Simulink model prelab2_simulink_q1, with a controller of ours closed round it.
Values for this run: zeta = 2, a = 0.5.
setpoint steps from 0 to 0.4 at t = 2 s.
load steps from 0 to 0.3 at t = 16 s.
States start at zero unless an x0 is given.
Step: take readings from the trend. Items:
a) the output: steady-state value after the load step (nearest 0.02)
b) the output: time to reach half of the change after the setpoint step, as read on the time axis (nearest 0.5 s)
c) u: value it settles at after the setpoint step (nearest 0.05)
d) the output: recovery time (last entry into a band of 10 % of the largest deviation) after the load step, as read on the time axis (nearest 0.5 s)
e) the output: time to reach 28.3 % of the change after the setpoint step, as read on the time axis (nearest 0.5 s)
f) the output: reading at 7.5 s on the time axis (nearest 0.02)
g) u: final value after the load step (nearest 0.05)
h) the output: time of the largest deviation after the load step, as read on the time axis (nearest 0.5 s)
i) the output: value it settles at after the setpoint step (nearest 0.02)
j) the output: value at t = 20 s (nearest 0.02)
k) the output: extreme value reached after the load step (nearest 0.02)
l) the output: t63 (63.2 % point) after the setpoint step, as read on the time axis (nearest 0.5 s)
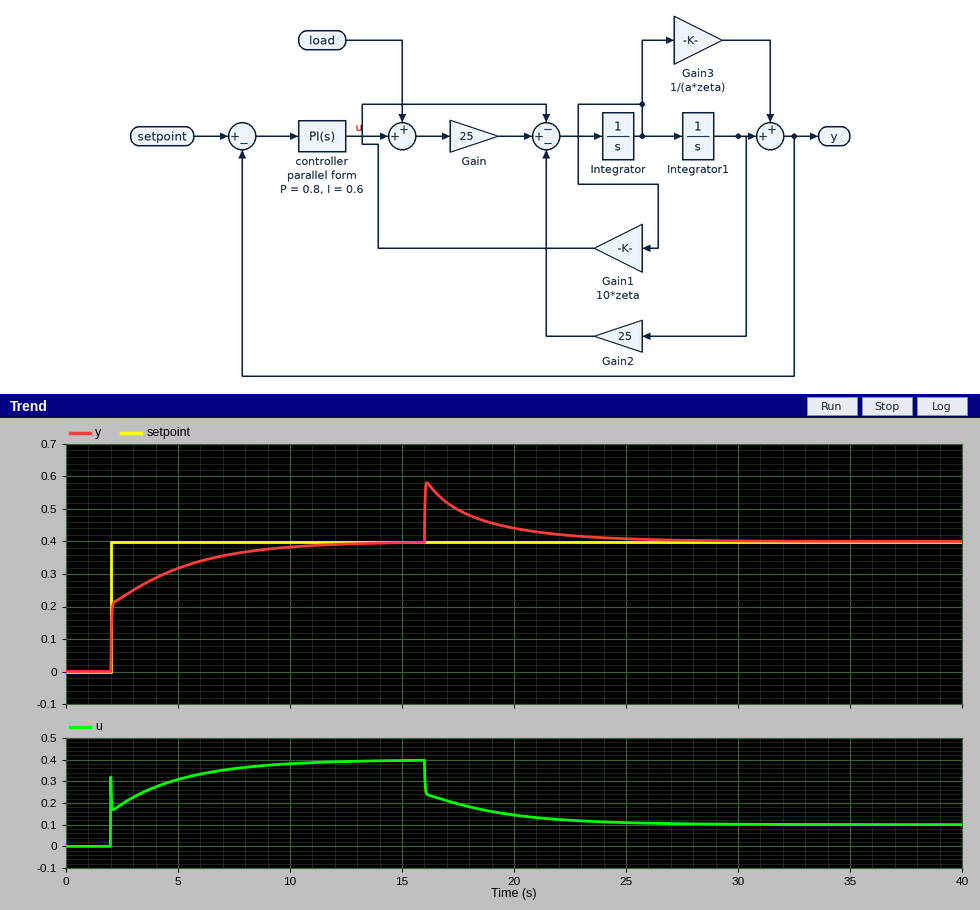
0.40
2.0 s
0.40
22.5 s
2.0 s
0.36
0.10
16.0 s
0.40
0.44
0.58
3.0 s
